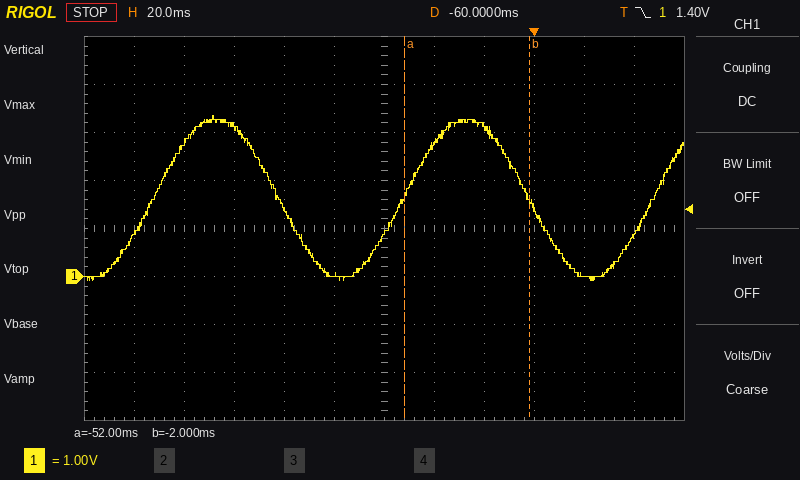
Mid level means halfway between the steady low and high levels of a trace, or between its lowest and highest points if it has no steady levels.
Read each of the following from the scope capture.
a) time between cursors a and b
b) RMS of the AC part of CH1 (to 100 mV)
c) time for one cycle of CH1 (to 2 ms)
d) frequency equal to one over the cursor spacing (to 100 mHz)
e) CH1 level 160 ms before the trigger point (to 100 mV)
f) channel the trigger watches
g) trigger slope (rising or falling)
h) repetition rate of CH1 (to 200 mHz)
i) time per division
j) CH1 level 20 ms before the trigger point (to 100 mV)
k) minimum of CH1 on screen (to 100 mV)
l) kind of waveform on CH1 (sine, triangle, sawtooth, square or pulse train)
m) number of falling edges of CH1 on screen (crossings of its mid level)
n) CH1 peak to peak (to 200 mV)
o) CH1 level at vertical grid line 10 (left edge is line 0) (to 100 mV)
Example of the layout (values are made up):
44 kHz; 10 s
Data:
50 ms; 1.2 V; 100 ms; 20.0 Hz; 900 mV; CH1; falling; 10.0 Hz; 20 ms; 3.1 V; -100 mV; sine; 2; 3.4 V; 0.0 V
